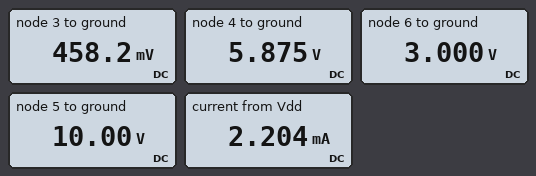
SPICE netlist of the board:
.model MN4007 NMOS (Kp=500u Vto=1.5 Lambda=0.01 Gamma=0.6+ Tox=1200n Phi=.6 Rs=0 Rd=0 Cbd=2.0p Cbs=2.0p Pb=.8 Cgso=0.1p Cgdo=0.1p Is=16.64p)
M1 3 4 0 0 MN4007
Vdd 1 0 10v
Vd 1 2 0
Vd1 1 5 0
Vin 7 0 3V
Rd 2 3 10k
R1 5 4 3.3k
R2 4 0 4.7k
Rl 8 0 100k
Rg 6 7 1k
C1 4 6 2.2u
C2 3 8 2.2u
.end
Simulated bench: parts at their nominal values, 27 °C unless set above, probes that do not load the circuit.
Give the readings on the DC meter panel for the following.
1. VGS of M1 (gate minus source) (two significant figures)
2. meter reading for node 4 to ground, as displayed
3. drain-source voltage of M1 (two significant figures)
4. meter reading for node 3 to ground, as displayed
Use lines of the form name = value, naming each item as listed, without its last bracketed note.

VGS of M1 (gate minus source) = 5.9 V
meter reading for node 4 to ground, as displayed = 5.875 V
drain-source voltage of M1 = 460 mV
meter reading for node 3 to ground, as displayed = 458.2 mV
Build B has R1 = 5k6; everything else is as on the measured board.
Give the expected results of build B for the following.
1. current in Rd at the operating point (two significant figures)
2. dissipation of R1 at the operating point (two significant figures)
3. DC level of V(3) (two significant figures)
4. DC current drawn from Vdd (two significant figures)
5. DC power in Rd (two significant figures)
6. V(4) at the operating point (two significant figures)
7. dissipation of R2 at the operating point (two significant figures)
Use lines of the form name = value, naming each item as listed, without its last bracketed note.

current in Rd at the operating point = 930 µA
dissipation of R1 at the operating point = 5.3 mW
DC level of V(3) = 680 mV
DC current drawn from Vdd = 1.9 mA
DC power in Rd = 8.7 mW
V(4) at the operating point = 4.6 V
dissipation of R2 at the operating point = 4.4 mW
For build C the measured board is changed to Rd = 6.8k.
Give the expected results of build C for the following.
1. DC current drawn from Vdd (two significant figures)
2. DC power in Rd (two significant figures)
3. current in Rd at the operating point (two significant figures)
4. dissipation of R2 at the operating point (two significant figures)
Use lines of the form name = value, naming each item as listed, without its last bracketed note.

DC current drawn from Vdd = 2.6 mA
DC power in Rd = 13 mW
current in Rd at the operating point = 1.4 mA
dissipation of R2 at the operating point = 7.3 mW
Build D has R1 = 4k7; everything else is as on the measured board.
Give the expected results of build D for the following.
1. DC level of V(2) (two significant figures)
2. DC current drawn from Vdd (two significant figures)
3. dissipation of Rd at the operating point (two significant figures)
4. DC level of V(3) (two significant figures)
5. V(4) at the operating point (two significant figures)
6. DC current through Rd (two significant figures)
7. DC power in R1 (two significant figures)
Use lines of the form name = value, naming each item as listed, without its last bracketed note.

DC level of V(2) = 10 V
DC current drawn from Vdd = 2.0 mA
dissipation of Rd at the operating point = 8.9 mW
DC level of V(3) = 580 mV
V(4) at the operating point = 5.0 V
DC current through Rd = 940 µA
DC power in R1 = 5.3 mW
